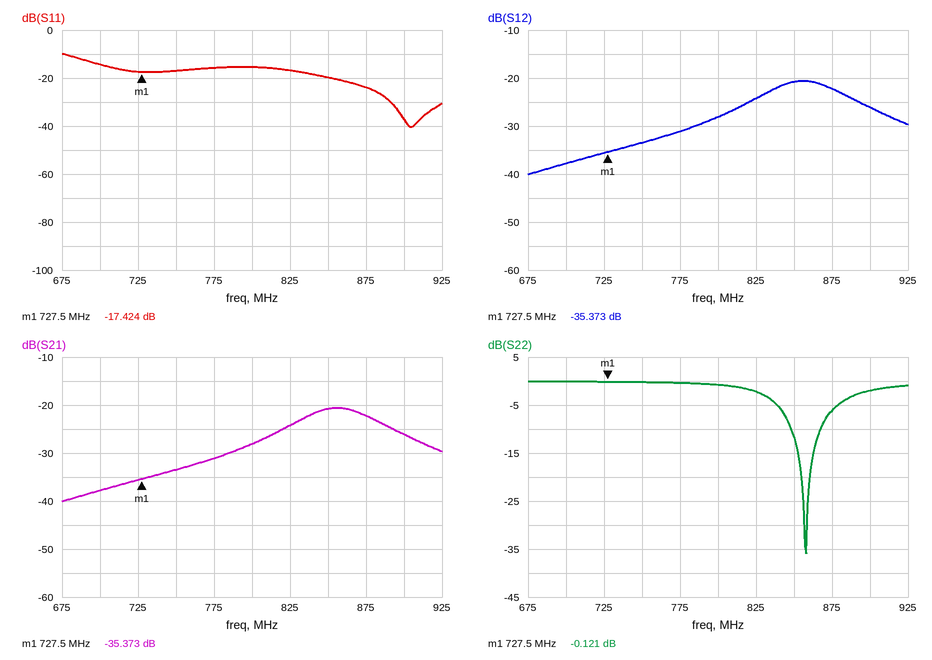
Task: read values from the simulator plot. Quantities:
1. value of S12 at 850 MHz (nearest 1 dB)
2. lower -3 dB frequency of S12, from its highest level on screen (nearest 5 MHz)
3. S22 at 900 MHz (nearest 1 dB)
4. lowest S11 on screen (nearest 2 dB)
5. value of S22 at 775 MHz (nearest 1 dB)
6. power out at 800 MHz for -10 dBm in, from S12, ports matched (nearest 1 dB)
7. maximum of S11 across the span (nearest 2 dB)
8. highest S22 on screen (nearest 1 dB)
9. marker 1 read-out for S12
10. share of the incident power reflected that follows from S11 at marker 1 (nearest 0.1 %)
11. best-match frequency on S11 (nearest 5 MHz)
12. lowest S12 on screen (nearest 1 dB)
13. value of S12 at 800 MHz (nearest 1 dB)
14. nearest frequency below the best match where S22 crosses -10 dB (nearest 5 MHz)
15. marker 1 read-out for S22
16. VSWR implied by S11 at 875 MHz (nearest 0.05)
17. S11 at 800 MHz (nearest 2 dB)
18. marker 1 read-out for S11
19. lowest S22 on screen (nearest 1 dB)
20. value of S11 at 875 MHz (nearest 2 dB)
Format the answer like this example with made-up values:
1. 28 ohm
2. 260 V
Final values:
1. -21 dB
2. 830 MHz
3. -2 dB
4. -40 dB
5. 0 dB
6. -38 dBm
7. -10 dB
8. 0 dB
9. -35.373 dB
10. 1.8 %
11. 905 MHz
12. -40 dB
13. -28 dB
14. 850 MHz
15. -0.121 dB
16. 1.15
17. -16 dB
18. -17.424 dB
19. -36 dB
20. -24 dB
